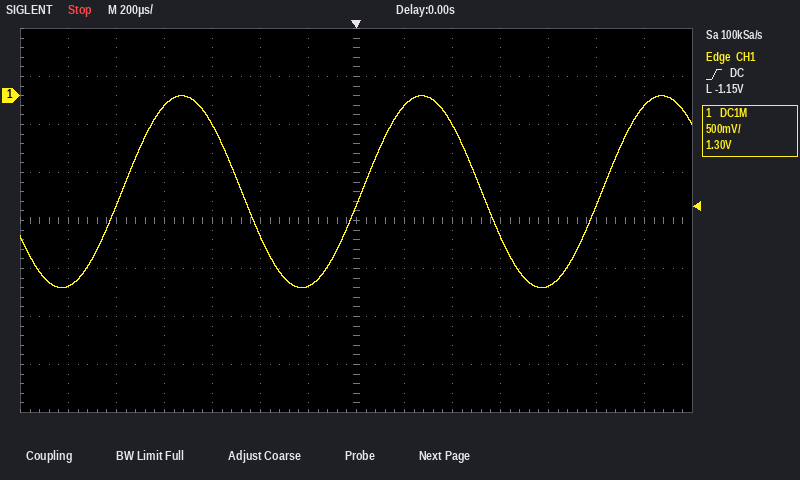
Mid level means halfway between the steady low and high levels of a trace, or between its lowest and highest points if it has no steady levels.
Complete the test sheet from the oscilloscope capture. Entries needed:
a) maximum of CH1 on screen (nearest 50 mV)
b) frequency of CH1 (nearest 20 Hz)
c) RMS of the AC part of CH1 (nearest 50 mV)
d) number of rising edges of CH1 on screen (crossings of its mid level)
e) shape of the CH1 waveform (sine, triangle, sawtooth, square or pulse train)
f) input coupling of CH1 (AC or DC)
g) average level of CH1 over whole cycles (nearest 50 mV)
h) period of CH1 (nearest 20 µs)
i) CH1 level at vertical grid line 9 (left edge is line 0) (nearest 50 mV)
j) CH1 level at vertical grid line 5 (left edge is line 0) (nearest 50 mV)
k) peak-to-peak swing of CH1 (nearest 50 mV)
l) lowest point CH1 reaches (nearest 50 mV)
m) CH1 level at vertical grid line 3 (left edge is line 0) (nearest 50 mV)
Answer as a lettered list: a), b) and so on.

a) 0 mV
b) 1.00 kHz
c) 700 mV
d) 3
e) sine
f) DC
g) -1.00 V
h) 1.00 ms
i) -300 mV
j) -1.45 V
k) 2.00 V
l) -2.00 V
m) -100 mV
